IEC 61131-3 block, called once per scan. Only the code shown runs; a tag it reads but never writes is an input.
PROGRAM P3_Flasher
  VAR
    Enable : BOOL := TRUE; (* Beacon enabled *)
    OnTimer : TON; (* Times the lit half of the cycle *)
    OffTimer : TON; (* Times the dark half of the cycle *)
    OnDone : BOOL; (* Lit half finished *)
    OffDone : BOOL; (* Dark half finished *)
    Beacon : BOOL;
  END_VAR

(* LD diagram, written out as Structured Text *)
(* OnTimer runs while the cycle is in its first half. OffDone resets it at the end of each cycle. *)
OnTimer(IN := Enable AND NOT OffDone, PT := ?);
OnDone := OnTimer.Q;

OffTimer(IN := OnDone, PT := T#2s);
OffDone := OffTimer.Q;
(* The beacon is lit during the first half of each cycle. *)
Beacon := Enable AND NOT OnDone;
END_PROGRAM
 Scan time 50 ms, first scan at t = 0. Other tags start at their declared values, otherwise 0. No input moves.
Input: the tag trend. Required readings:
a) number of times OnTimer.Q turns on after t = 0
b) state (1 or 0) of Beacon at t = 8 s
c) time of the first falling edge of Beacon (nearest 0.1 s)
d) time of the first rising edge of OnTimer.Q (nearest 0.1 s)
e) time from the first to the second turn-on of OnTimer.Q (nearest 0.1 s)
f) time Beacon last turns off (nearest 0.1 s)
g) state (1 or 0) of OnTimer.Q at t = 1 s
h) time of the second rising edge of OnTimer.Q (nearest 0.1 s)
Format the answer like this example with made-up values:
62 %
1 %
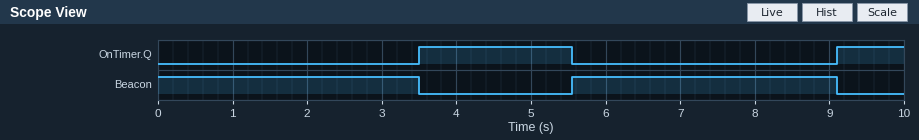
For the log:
2
1
3.5 s
3.5 s
5.6 s
9.1 s
0
9.1 s
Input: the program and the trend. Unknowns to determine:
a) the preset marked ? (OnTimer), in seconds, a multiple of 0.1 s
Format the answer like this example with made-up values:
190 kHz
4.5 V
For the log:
3.5 s
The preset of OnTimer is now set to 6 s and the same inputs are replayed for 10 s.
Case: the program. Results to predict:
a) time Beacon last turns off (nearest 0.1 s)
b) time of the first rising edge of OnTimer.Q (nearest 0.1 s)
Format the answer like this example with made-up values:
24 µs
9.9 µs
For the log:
6.0 s
6.0 s
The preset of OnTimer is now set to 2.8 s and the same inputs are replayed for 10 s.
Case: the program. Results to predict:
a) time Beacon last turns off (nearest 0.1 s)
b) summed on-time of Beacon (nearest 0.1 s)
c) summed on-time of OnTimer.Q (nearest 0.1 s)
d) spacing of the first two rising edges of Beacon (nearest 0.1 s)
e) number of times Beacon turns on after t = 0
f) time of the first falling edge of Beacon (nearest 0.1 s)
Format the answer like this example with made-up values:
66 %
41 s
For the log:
7.7 s
5.9 s
4.1 s
4.9 s
2
2.8 s
